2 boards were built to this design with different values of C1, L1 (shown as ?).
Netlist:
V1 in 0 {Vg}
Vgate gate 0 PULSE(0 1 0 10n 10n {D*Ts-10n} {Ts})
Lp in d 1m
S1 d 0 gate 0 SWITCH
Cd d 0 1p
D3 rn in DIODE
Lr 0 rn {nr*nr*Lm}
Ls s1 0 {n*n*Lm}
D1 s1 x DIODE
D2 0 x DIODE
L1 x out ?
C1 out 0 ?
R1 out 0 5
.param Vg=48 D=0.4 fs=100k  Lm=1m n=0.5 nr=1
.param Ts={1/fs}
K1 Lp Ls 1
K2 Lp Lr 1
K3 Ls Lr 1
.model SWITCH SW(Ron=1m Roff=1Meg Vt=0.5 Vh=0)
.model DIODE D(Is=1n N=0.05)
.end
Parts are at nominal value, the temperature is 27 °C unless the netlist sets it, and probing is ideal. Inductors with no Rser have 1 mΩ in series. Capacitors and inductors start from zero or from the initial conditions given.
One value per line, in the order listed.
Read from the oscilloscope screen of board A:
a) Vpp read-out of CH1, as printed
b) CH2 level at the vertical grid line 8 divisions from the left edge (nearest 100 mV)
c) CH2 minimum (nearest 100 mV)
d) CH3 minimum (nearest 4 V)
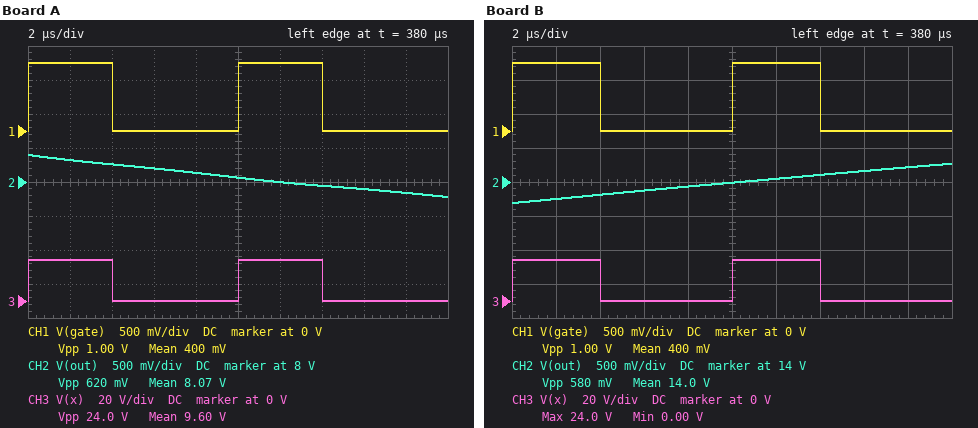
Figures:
1.00 V
7.9 V
7.8 V
0 V
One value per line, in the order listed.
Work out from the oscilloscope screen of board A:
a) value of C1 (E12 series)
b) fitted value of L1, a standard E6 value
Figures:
33 µF
150 µH
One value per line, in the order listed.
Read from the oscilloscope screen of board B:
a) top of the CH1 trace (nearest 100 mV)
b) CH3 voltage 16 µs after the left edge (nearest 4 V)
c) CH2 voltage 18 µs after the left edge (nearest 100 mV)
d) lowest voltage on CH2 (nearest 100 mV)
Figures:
1.0 V
0 V
14.2 V
13.7 V
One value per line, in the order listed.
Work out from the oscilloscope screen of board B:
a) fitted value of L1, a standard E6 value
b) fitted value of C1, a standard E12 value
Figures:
220 µH
120 µF
